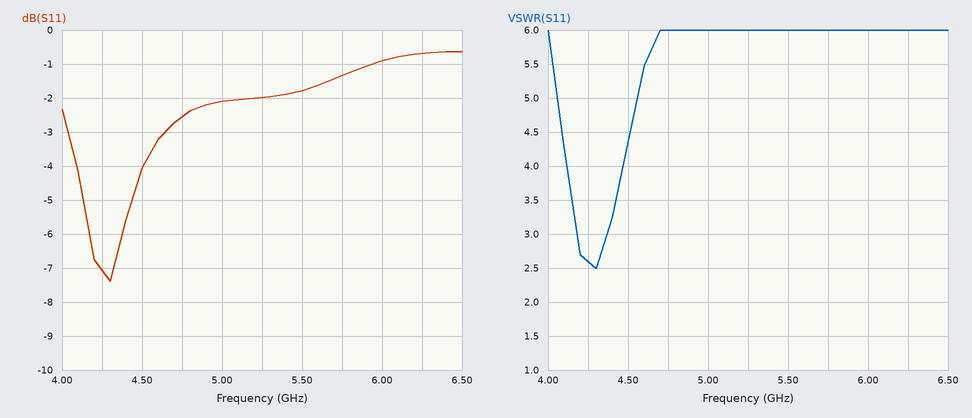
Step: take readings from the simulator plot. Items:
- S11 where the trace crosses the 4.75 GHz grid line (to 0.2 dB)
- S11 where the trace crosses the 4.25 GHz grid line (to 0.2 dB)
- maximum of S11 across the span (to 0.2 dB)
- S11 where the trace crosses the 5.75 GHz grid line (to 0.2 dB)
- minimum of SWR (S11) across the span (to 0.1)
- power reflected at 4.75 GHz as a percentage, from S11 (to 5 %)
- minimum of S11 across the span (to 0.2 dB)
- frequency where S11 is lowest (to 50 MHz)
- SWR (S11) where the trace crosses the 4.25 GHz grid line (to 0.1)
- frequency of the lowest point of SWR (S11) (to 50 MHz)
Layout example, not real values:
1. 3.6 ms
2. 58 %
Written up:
1. -2.6 dB
2. -7.0 dB
3. -0.6 dB
4. -1.4 dB
5. 2.5
6. 55 %
7. -7.4 dB
8. 4.30 GHz
9. 2.6
10. 4.30 GHz
